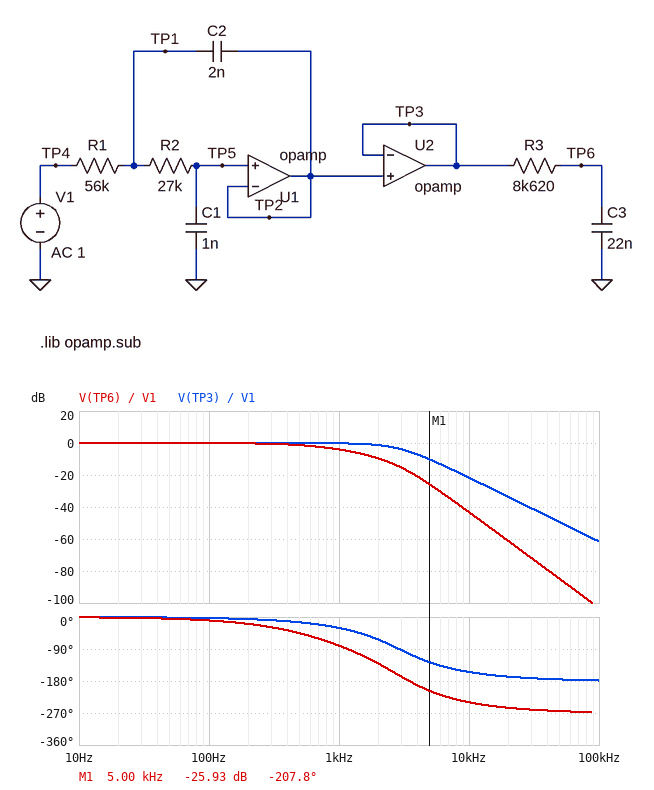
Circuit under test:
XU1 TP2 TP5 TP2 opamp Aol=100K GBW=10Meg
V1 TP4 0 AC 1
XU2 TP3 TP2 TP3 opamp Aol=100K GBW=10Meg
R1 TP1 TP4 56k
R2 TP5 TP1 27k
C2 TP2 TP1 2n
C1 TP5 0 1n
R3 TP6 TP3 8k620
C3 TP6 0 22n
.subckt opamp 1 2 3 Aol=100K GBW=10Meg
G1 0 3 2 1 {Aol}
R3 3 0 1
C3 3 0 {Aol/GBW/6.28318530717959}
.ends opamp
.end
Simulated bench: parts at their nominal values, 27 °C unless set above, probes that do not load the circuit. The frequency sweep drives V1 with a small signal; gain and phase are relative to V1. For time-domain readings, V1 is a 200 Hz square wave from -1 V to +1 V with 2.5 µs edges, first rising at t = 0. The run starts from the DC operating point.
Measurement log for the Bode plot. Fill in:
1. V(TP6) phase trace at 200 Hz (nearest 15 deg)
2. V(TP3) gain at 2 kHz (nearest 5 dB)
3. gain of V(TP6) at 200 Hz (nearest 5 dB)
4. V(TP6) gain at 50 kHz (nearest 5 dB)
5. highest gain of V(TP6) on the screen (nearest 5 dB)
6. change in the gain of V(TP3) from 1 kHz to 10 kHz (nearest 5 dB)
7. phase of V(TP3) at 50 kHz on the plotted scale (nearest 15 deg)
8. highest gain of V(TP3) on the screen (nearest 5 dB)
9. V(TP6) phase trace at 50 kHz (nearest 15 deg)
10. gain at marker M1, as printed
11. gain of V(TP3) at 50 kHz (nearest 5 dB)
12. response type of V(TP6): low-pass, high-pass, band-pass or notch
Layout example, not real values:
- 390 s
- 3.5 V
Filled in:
- -15 deg
- 0 dB
- 0 dB
- -85 dB
- 0 dB
- -20 dB
- -180 deg
- 0 dB
- -270 deg
- -25.93 dB
- -50 dB
- low-pass
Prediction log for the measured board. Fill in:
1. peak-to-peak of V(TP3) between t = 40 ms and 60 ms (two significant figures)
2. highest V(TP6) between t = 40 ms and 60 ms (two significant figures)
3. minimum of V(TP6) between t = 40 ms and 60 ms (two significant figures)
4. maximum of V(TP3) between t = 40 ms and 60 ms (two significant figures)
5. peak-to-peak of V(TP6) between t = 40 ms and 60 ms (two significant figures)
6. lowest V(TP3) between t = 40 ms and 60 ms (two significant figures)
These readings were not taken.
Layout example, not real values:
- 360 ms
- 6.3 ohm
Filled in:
- 2.1 V
- 1.0 V
- -1.0 V
- 1.1 V
- 2.0 V
- -1.1 V
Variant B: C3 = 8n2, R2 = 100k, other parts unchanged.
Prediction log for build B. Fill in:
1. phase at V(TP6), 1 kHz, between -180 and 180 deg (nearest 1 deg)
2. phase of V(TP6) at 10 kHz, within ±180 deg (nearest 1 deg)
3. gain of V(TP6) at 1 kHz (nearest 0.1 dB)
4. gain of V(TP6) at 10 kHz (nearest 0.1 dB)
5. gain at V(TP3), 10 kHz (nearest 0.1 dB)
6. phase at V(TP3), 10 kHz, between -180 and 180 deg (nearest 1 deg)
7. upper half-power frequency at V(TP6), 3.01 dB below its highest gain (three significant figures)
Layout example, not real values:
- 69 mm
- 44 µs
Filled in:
- -84 deg
- 115 deg
- -1.8 dB
- -46.1 dB
- -32.9 dB
- -167 deg
- 1.22 kHz
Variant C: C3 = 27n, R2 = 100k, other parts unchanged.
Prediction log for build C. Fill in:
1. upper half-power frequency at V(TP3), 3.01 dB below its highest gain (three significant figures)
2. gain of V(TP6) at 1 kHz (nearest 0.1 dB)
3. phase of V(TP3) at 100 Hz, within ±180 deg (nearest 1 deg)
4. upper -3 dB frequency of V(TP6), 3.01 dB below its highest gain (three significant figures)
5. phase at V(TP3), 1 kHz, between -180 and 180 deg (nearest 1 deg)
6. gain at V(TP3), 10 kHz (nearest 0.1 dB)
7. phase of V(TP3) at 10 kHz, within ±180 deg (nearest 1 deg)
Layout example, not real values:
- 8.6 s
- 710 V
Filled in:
- 1.44 kHz
- -6.0 dB
- -6 deg
- 641 Hz
- -60 deg
- -32.9 dB
- -167 deg
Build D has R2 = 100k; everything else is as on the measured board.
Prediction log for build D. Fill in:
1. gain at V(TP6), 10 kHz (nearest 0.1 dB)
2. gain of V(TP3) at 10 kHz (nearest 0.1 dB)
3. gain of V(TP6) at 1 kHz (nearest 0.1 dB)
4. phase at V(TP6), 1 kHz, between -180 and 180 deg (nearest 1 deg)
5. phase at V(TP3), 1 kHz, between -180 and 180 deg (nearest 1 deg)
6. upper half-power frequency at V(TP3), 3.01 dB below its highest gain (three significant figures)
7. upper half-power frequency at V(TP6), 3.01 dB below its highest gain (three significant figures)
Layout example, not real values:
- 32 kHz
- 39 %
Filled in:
- -54.5 dB
- -32.9 dB
- -4.9 dB
- -110 deg
- -60 deg
- 1.44 kHz
- 754 Hz
